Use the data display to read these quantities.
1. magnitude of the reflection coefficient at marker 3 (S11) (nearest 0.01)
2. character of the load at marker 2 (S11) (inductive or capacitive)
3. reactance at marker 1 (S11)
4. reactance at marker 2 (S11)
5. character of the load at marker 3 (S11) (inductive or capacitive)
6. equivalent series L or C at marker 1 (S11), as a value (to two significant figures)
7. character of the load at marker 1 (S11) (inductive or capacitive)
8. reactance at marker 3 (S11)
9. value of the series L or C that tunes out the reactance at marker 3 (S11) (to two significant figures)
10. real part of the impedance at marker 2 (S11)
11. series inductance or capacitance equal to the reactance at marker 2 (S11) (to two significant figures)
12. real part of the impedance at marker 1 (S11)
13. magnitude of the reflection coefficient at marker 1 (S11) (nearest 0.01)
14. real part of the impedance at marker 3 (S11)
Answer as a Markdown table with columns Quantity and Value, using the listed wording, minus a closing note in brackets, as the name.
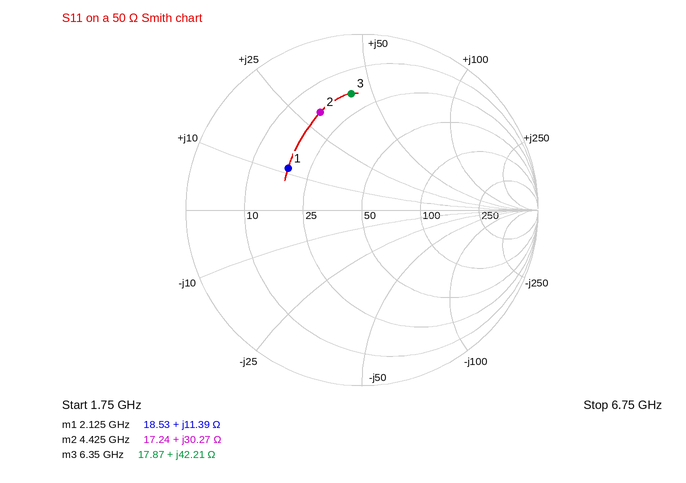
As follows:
| Quantity | Value |
|---|---|
| magnitude of the reflection coefficient at marker 3 (S11) | 0.66 |
| character of the load at marker 2 (S11) | inductive |
| reactance at marker 1 | +11.39 Ω |
| reactance at marker 2 | +30.27 Ω |
| character of the load at marker 3 (S11) | inductive |
| equivalent series L or C at marker 1 (S11), as a value | 850 pH |
| character of the load at marker 1 (S11) | inductive |
| reactance at marker 3 | +42.21 Ω |
| value of the series L or C that tunes out the reactance at marker 3 (S11) | 590 fF |
| real part of the impedance at marker 2 | 17.24 Ω |
| series inductance or capacitance equal to the reactance at marker 2 (S11) | 1.1 nH |
| real part of the impedance at marker 1 | 18.53 Ω |
| magnitude of the reflection coefficient at marker 1 (S11) | 0.48 |
| real part of the impedance at marker 3 | 17.87 Ω |
